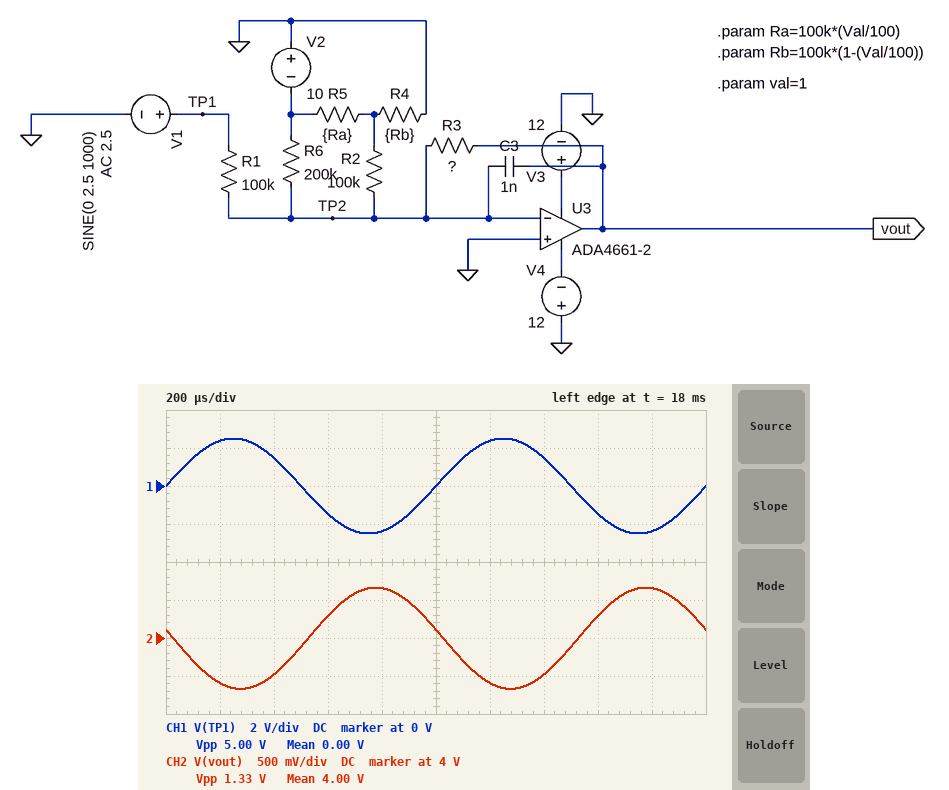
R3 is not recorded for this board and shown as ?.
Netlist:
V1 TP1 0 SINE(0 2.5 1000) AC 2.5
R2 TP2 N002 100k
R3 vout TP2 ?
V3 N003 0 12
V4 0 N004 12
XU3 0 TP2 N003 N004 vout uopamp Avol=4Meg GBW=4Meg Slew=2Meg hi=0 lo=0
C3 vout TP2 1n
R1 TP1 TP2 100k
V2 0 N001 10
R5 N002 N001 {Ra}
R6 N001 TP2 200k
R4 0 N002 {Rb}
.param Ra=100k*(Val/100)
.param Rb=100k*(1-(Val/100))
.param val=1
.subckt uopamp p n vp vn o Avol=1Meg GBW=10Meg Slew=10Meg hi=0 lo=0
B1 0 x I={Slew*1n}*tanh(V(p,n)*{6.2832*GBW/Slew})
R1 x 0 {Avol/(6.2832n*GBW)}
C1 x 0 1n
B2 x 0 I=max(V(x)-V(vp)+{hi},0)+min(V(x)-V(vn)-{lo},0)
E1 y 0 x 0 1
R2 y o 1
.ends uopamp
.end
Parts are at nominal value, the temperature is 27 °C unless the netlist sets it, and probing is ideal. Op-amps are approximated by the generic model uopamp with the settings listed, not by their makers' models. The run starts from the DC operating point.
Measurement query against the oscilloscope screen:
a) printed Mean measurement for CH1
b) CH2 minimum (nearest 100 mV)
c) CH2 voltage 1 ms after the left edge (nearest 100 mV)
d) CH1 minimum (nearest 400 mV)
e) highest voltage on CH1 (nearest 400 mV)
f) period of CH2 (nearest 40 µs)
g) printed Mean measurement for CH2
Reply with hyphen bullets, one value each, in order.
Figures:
- 0.00 V
- 3.3 V
- 4.1 V
- -2.4 V
- 2.4 V
- 1.00 ms
- 4.00 V
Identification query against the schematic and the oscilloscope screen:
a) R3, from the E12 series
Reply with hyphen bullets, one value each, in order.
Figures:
- 27 kΩ
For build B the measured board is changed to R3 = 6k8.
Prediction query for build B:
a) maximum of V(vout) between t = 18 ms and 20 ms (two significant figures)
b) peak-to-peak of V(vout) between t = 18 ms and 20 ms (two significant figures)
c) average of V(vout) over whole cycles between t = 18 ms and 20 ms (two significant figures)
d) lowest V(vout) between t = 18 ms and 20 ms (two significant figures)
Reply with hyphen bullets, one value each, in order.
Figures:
- 1.2 V
- 340 mV
- 1.0 V
- 840 mV
